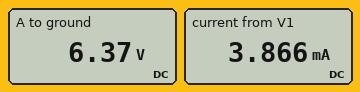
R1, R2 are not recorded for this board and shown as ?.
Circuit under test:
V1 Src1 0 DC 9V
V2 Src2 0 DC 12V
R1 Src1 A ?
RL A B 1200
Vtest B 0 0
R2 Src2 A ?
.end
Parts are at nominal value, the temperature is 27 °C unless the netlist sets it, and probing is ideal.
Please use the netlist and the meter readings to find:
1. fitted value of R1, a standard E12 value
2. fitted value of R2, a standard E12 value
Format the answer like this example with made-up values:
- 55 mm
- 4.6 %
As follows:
- 680 Ω
- 3.9 kΩ
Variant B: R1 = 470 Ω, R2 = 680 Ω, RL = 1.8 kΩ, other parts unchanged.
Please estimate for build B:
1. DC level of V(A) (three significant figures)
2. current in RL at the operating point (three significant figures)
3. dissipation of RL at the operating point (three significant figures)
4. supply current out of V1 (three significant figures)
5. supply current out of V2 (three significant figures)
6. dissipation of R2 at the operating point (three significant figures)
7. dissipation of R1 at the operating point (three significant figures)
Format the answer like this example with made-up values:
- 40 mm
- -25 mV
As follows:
- 8.86 V
- 4.92 mA
- 43.6 mW
- 301 µA
- 4.62 mA
- 14.5 mW
- 42.7 µW
